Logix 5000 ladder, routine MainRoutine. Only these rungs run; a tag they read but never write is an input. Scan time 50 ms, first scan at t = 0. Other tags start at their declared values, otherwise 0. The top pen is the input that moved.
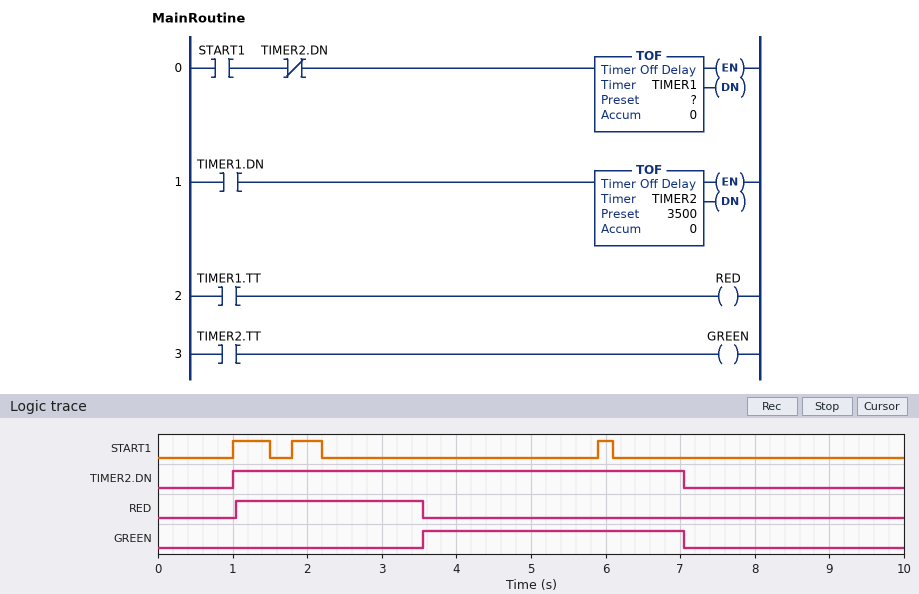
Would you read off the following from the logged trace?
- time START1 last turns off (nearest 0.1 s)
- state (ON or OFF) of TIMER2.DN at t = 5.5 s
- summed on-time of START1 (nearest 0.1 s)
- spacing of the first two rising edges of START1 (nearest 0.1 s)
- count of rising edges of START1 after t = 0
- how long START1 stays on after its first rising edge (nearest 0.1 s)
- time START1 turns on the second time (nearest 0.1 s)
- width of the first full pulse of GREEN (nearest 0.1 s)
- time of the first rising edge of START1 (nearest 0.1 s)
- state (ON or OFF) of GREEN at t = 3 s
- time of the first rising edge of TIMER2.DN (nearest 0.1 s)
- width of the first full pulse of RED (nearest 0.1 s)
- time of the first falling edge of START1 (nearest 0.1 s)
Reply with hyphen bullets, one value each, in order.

- 6.1 s
- ON
- 1.1 s
- 0.8 s
- 3
- 0.5 s
- 1.8 s
- 3.5 s
- 1.0 s
- OFF
- 1.0 s
- 2.5 s
- 1.5 s
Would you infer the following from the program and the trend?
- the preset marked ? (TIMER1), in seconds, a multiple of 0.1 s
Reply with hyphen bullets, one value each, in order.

- 2.5 s
